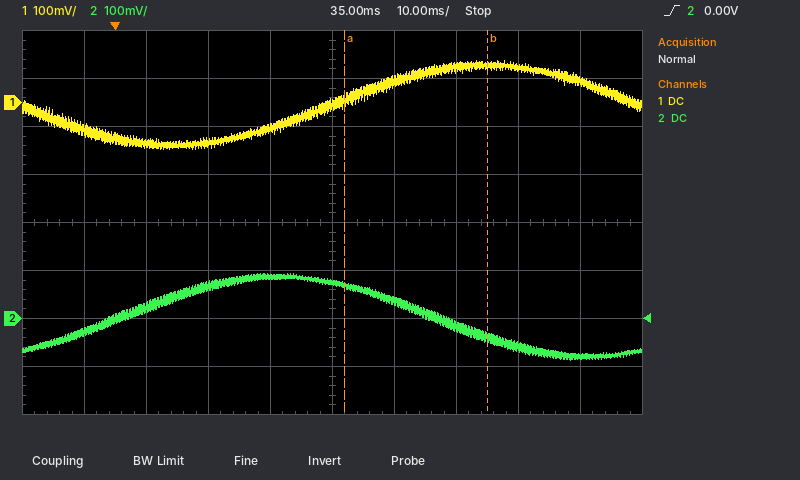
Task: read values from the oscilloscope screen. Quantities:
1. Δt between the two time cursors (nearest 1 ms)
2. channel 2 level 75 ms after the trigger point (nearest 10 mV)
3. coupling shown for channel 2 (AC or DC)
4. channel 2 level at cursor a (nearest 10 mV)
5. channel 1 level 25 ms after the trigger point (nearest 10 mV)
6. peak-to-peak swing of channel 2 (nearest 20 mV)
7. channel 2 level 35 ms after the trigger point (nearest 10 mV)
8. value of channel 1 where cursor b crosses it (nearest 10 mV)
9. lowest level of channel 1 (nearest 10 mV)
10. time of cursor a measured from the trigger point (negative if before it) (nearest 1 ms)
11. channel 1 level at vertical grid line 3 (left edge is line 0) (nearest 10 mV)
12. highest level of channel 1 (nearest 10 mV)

23 ms
-80 mV
DC
70 mV
-50 mV
180 mV
80 mV
80 mV
-100 mV
+37 ms
-80 mV
90 mV
